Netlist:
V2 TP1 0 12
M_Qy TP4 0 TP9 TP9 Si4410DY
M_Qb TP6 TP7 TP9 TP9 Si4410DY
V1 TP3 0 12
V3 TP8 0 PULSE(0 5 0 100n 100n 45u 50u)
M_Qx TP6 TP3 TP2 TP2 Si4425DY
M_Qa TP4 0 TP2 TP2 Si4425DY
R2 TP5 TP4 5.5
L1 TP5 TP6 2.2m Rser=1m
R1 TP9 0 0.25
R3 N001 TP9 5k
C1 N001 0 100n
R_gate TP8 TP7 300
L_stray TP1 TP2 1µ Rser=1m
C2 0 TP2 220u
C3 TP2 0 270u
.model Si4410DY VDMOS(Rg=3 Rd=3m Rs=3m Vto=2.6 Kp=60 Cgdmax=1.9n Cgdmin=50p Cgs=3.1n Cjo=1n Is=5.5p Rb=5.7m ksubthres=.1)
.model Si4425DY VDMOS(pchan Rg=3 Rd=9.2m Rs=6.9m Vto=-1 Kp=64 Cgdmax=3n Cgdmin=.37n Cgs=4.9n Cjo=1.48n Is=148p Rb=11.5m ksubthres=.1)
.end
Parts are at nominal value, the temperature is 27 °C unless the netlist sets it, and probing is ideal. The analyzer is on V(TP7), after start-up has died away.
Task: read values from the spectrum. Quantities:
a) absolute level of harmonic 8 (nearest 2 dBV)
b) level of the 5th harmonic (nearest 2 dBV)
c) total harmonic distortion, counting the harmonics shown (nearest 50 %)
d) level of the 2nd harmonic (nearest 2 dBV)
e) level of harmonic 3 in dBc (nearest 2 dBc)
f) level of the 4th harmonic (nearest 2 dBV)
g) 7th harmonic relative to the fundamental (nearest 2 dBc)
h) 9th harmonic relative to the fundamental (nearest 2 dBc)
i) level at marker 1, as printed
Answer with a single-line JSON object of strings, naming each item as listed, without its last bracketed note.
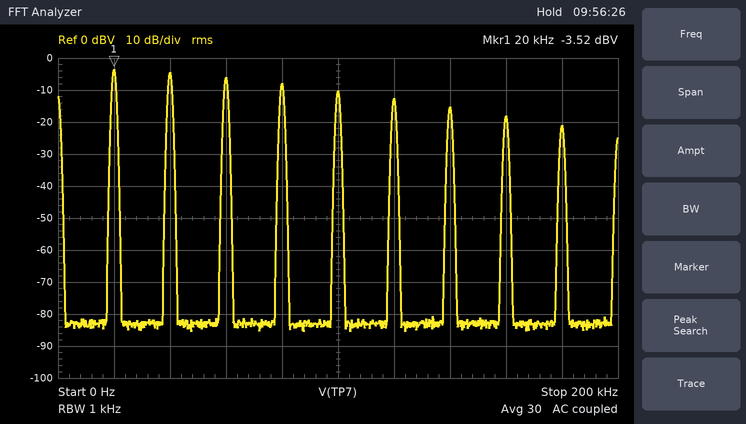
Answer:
{"absolute level of harmonic 8": "-18 dBV", "level of the 5th harmonic": "-10 dBV", "total harmonic distortion, counting the harmonics shown": "150 %", "level of the 2nd harmonic": "-4 dBV", "level of harmonic 3 in dBc": "-2 dBc", "level of the 4th harmonic": "-8 dBV", "7th harmonic relative to the fundamental": "-12 dBc", "9th harmonic relative to the fundamental": "-18 dBc", "level at marker 1, as printed": "-3.52 dBV"}
